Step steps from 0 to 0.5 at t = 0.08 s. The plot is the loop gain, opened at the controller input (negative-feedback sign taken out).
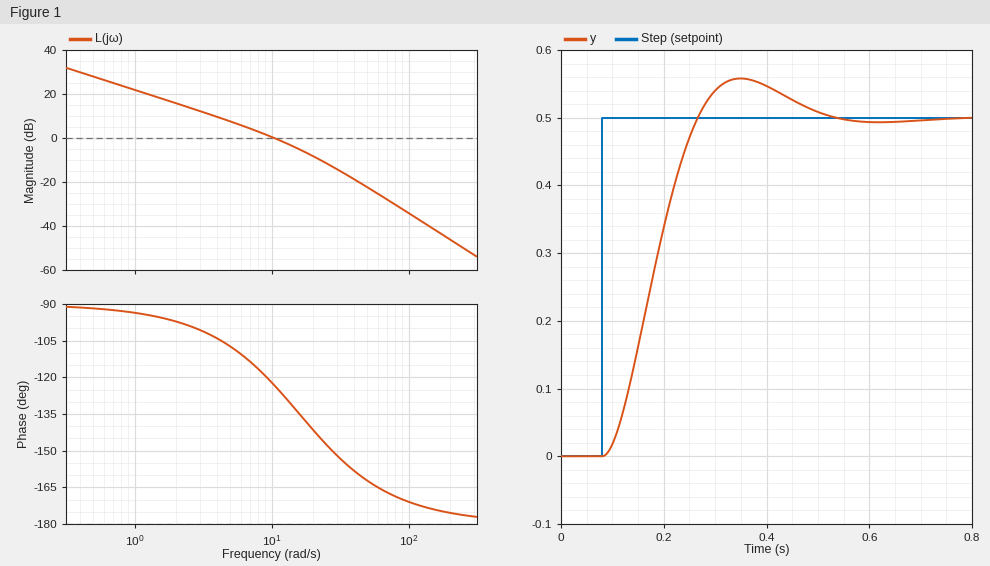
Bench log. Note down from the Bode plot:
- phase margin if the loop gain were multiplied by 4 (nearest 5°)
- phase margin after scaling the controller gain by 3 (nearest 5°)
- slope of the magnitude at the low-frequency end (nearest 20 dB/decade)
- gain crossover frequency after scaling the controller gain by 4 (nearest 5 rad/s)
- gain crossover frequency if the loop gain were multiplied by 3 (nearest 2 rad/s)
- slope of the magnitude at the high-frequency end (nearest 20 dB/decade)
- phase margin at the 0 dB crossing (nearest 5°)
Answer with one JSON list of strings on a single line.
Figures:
["30°", "35°", "-20 dB/decade", "25 rad/s", "22 rad/s", "-40 dB/decade", "55°"]
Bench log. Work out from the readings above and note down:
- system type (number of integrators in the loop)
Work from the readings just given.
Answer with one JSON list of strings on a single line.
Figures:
["1"]
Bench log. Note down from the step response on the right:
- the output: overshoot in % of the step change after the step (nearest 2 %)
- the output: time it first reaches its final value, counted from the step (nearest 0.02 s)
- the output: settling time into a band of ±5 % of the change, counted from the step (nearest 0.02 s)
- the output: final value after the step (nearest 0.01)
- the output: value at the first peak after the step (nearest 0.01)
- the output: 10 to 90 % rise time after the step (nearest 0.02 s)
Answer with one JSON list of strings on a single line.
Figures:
["12 %", "0.18 s", "0.38 s", "0.50", "0.56", "0.12 s"]
